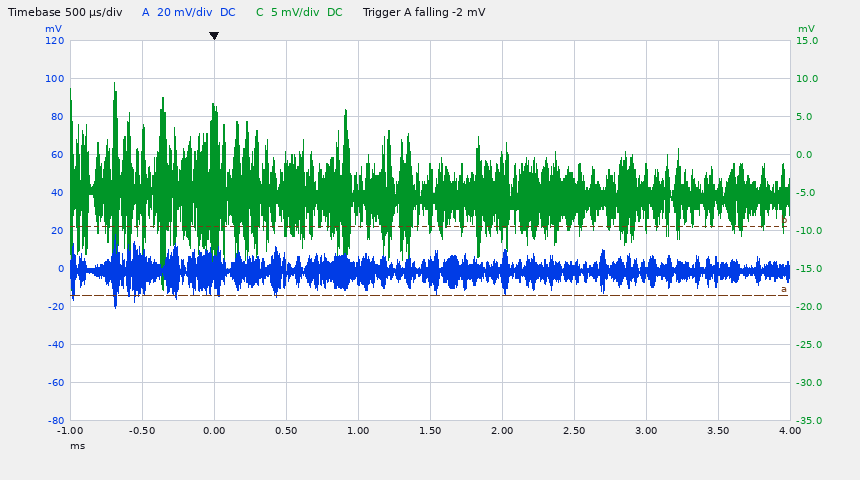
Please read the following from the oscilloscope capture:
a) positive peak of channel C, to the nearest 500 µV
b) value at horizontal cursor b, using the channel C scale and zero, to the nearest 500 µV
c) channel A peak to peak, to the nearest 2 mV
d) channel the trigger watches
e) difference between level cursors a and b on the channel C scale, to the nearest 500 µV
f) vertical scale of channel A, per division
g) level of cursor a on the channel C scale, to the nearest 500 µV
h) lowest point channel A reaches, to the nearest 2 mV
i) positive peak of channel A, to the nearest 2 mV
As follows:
9.5 mV
-9.5 mV
38 mV
channel A
9.0 mV
20 mV
-18.5 mV
-20 mV
18 mV
